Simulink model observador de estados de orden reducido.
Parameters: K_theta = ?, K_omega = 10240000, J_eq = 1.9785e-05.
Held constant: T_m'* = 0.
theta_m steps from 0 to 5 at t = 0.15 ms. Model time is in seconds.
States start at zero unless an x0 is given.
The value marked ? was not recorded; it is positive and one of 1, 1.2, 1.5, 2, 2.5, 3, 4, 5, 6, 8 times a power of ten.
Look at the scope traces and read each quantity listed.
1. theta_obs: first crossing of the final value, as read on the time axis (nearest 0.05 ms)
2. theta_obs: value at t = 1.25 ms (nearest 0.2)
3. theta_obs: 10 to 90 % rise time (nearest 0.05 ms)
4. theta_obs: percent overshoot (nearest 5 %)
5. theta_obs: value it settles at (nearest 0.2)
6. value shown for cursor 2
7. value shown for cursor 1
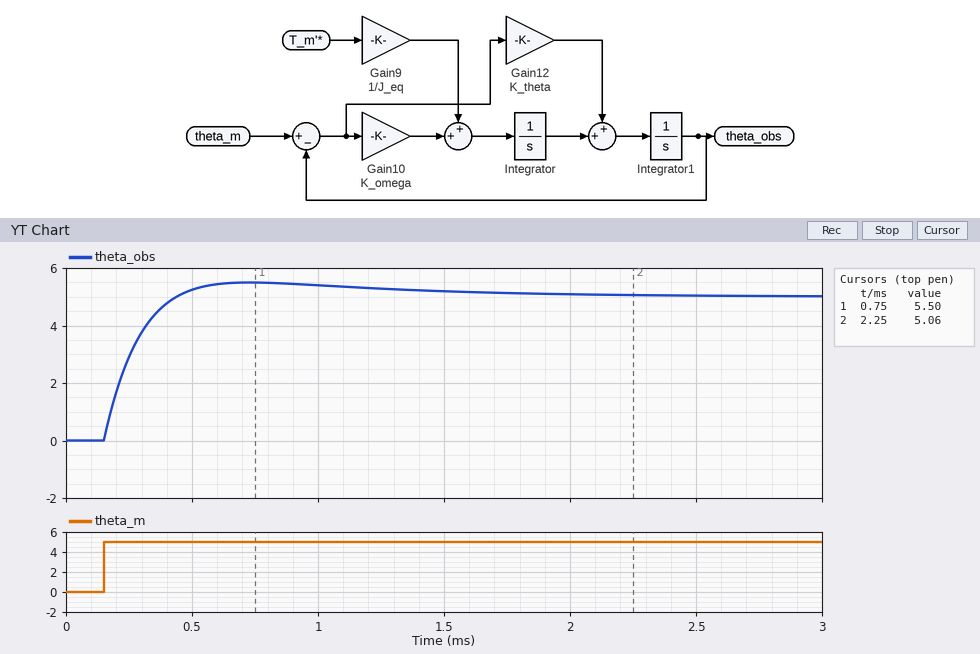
0.45 ms
5.2
0.20 ms
10 %
5.0
5.06
5.50
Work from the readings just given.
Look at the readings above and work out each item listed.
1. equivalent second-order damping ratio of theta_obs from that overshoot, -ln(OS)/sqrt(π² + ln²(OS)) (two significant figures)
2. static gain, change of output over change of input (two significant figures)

0.59
1.0
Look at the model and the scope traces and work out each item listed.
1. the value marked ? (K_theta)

8000
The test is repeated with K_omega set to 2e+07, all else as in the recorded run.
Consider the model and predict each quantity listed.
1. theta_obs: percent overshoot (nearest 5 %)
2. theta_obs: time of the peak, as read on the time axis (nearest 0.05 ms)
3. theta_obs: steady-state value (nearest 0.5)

15 %
0.60 ms
5.0
